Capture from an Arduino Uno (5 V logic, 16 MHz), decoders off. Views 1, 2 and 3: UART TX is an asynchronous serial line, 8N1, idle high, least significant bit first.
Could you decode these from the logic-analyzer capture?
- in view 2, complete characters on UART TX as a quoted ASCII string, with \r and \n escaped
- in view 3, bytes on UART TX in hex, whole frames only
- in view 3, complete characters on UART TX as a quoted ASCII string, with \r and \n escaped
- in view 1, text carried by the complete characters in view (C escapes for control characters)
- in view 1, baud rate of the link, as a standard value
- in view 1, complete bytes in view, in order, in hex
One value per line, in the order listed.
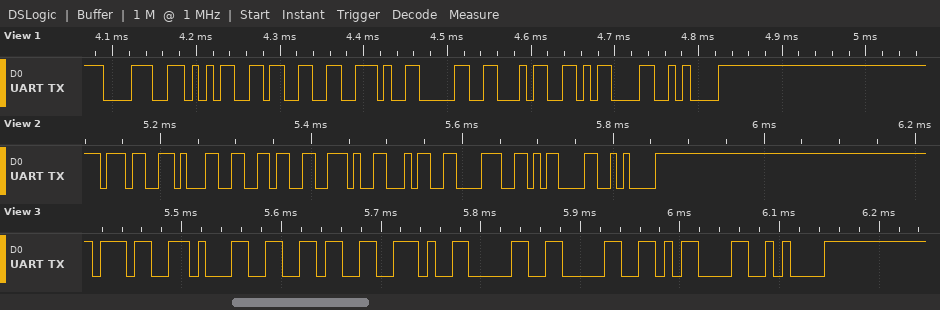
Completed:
"716.48\r\n"
37 31 36 2E 30 30 0D 0A
"716.00\r\n"
"853.04\r\n"
115200 baud
0x38 0x35 0x33 0x2E 0x30 0x34 0x0D 0x0A
